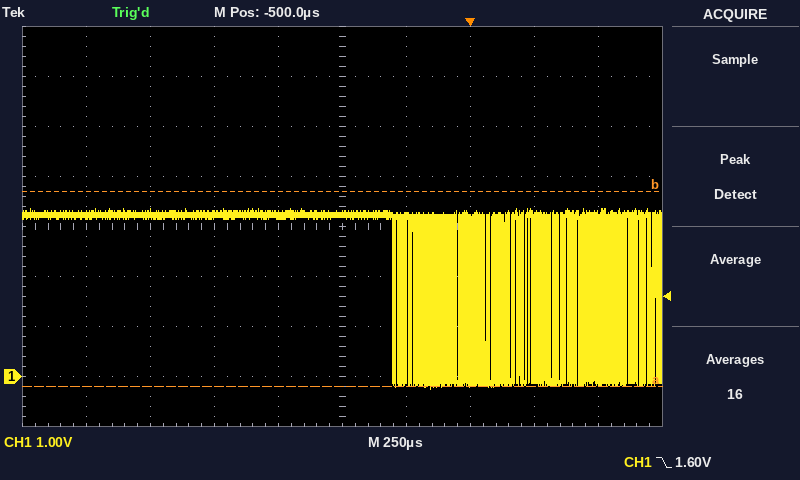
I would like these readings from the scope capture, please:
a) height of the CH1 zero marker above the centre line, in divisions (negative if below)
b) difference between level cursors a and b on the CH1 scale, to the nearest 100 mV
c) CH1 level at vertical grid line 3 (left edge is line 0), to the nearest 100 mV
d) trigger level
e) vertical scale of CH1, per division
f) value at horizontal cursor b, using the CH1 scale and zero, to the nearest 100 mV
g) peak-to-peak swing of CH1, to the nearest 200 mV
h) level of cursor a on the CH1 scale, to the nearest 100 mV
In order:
-3.0 div
3.9 V
3.2 V
1.60 V
1 V
3.7 V
3.6 V
-200 mV
